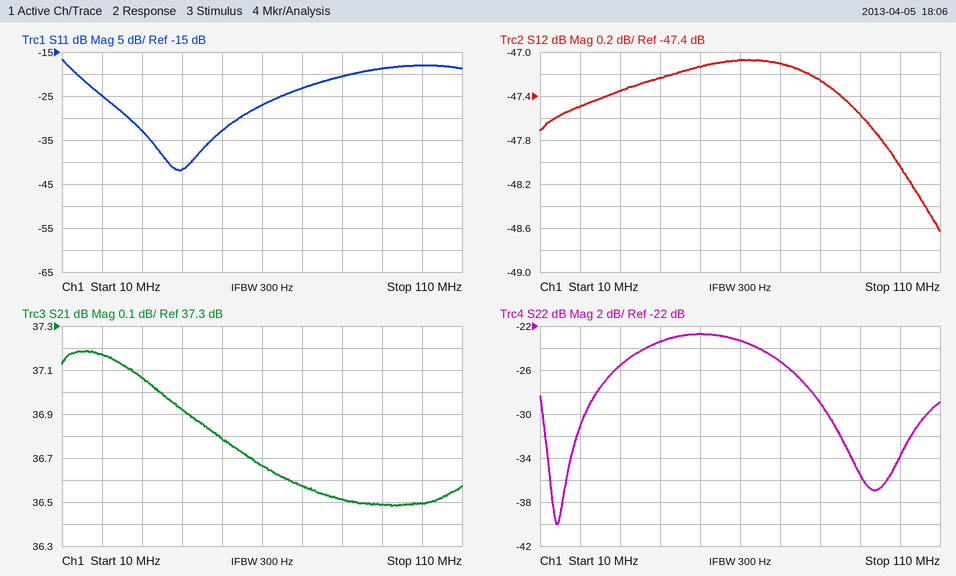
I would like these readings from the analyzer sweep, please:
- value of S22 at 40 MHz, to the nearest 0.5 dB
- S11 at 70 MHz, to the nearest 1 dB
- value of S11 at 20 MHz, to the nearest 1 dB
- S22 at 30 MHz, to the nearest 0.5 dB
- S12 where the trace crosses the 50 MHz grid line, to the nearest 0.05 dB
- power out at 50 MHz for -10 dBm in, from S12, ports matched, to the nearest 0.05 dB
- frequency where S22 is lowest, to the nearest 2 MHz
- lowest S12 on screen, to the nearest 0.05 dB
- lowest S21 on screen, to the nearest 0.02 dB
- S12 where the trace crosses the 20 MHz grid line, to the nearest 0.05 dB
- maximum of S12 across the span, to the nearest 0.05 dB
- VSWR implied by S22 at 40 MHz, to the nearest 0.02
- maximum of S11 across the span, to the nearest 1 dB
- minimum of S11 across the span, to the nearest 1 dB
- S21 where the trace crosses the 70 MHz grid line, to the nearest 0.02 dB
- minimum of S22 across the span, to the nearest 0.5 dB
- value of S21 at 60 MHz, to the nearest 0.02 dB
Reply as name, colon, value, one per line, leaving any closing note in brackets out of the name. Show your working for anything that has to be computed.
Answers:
value of S22 at 40 MHz, to the nearest 0.5 dB: -23.5 dB
S11 at 70 MHz, to the nearest 1 dB: -23 dB
value of S11 at 20 MHz, to the nearest 1 dB: -25 dB
S22 at 30 MHz, to the nearest 0.5 dB: -25.5 dB
S12 where the trace crosses the 50 MHz grid line, to the nearest 0.05 dB: -47.15 dB
power out at 50 MHz for -10 dBm in, from S12, ports matched, to the nearest 0.05 dB: -10 dBm + (-47.15 dB) = -57.15 dBm
frequency where S22 is lowest, to the nearest 2 MHz: 14 MHz
lowest S12 on screen, to the nearest 0.05 dB: -48.65 dB
lowest S21 on screen, to the nearest 0.02 dB: 36.48 dB
S12 where the trace crosses the 20 MHz grid line, to the nearest 0.05 dB: -47.50 dB
maximum of S12 across the span, to the nearest 0.05 dB: -47.05 dB
VSWR implied by S22 at 40 MHz, to the nearest 0.02: |Γ| = 10^(-23.5/20) = 0.0668; VSWR = (1 + 0.0668)/(1 − 0.0668) ≈ 1.14
maximum of S11 across the span, to the nearest 1 dB: -17 dB
minimum of S11 across the span, to the nearest 1 dB: -42 dB
S21 where the trace crosses the 70 MHz grid line, to the nearest 0.02 dB: 36.58 dB
minimum of S22 across the span, to the nearest 0.5 dB: -40.0 dB
value of S21 at 60 MHz, to the nearest 0.02 dB: 36.66 dB
